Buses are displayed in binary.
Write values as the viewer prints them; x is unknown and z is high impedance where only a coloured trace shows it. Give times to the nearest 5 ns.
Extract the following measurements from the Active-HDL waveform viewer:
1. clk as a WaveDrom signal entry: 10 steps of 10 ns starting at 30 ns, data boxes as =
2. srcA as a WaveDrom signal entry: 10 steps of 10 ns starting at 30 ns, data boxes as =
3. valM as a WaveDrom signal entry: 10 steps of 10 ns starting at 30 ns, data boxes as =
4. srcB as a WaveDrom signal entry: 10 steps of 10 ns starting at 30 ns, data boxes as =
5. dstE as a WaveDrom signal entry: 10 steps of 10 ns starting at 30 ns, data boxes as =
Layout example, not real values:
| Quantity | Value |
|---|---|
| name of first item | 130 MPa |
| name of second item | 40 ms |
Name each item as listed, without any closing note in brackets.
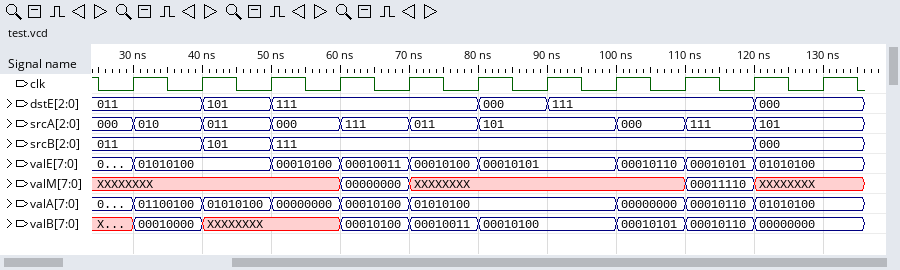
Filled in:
| Quantity | Value |
|---|---|
| clk as a WaveDrom signal entry: 10 steps of 10 ns starting at 30 ns, data boxes as = | {name: 'clk', wave: 'p.........'} |
| srcA as a WaveDrom signal entry: 10 steps of 10 ns starting at 30 ns, data boxes as = | {name: 'srcA', wave: '======.===', data: '010 011 000 111 011 101 000 111 101'} |
| valM as a WaveDrom signal entry: 10 steps of 10 ns starting at 30 ns, data boxes as = | {name: 'valM', wave: 'x..=x...=x', data: '00000000 00011110'} |
| srcB as a WaveDrom signal entry: 10 steps of 10 ns starting at 30 ns, data boxes as = | {name: 'srcB', wave: '===......=', data: '011 101 111 000'} |
| dstE as a WaveDrom signal entry: 10 steps of 10 ns starting at 30 ns, data boxes as = | {name: 'dstE', wave: '===..==..=', data: '011 101 111 000 111 000'} |
